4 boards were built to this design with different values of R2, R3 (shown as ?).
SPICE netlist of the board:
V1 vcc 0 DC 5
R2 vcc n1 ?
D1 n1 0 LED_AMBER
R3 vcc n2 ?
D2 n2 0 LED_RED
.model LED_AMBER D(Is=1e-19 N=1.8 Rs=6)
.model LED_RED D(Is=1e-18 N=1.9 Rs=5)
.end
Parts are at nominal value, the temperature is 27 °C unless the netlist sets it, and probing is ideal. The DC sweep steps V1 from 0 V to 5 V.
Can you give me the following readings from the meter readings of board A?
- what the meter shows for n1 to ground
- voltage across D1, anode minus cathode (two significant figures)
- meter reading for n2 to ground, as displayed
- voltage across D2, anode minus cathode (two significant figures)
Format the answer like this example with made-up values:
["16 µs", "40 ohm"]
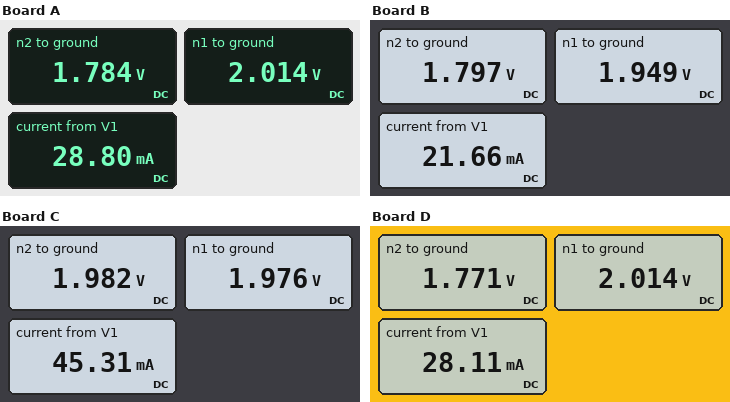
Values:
["2.014 V", "2.0 V", "1.784 V", "1.8 V"]
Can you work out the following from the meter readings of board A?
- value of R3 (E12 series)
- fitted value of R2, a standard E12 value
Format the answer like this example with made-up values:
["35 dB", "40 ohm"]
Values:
["820 Ω", "120 Ω"]
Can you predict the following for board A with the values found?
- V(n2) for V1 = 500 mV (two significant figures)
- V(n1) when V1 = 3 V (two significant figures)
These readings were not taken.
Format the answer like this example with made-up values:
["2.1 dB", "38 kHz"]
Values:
["500 mV", "1.9 V"]
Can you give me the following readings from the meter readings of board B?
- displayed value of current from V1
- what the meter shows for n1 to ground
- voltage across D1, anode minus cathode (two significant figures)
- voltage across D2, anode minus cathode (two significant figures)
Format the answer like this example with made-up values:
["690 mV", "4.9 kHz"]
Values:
["21.66 mA", "1.949 V", "1.9 V", "1.8 V"]
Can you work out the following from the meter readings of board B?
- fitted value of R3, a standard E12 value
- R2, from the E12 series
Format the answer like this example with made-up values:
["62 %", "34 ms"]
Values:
["680 Ω", "180 Ω"]
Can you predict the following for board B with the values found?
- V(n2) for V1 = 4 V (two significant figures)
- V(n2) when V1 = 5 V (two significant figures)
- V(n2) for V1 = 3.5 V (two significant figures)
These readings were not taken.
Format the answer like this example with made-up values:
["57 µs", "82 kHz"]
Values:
["1.8 V", "1.8 V", "1.8 V"]
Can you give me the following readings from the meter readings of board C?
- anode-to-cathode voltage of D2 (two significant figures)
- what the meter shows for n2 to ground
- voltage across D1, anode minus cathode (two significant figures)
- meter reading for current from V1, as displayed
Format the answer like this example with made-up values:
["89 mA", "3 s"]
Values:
["2.0 V", "1.982 V", "2.0 V", "45.31 mA"]
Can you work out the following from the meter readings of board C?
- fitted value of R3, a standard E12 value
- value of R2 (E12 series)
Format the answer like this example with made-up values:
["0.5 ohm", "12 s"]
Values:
["120 Ω", "150 Ω"]
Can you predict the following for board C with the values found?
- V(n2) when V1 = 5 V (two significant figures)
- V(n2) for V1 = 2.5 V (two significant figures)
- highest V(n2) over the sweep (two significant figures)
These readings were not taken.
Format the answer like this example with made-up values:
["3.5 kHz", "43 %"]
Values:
["2.0 V", "1.8 V", "2.0 V"]
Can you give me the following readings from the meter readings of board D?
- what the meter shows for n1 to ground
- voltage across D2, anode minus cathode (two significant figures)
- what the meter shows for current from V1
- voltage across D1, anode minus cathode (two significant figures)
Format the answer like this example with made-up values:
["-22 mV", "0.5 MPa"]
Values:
["2.014 V", "1.8 V", "28.11 mA", "2.0 V"]
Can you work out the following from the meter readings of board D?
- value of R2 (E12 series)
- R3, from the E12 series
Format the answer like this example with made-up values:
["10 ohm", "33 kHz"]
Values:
["120 Ω", "1 kΩ"]
